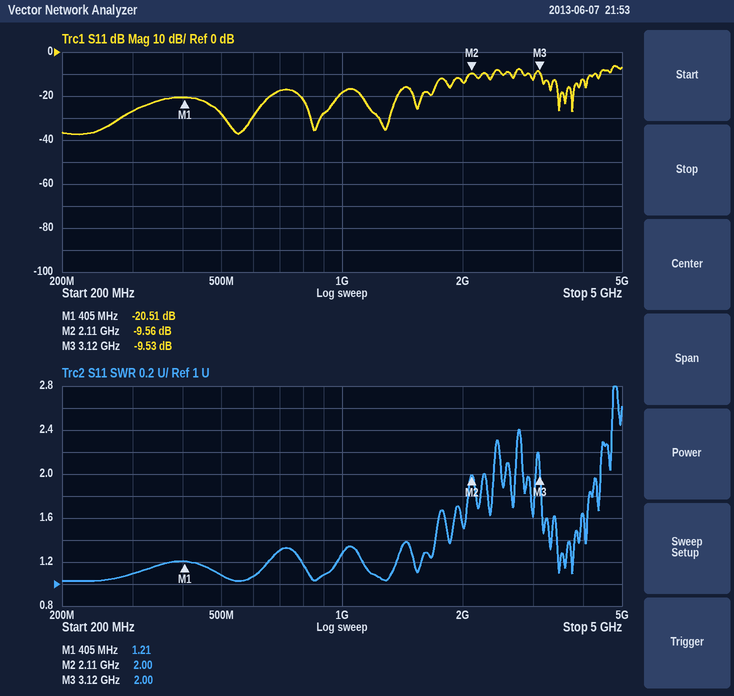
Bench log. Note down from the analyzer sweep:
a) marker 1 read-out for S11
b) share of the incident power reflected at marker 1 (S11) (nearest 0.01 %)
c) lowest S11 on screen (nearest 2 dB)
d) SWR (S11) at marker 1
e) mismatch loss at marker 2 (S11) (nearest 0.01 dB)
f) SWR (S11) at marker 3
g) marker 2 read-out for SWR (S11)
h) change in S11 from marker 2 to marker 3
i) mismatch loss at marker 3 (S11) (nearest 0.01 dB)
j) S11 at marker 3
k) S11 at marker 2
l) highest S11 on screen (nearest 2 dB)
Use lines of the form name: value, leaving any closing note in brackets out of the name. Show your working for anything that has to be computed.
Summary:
marker 1 read-out for S11: -20.51 dB
share of the incident power reflected at marker 1 (S11): 10^(-20.51/10) ≈ 0.89 %
lowest S11 on screen: -38 dB
SWR (S11) at marker 1: 1.21
mismatch loss at marker 2 (S11): −10 log10(1 − 10^(-9.56/10)) ≈ 0.51 dB
SWR (S11) at marker 3: 2.00
marker 2 read-out for SWR: 2.00
change in S11 from marker 2 to marker 3: -9.53 − (-9.56) = 0.03 dB
mismatch loss at marker 3 (S11): −10 log10(1 − 10^(-9.53/10)) ≈ 0.51 dB
S11 at marker 3: -9.53 dB
S11 at marker 2: -9.56 dB
highest S11 on screen: -6 dB
